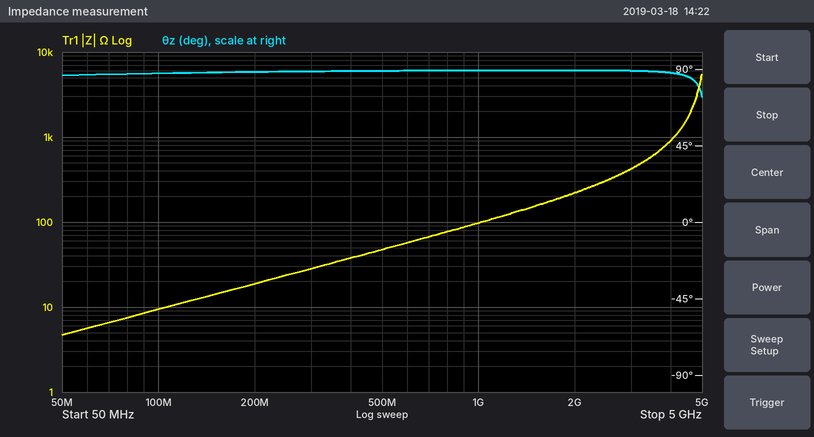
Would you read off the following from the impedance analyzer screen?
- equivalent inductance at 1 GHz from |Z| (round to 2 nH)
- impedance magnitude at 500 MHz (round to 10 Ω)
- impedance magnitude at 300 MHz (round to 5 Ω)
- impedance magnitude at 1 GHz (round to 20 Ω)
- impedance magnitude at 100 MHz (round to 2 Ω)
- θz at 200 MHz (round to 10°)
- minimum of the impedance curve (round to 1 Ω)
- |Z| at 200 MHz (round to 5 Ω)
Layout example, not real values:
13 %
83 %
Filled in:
16 nH
50 Ω
30 Ω
100 Ω
10 Ω
90°
5 Ω
20 Ω
